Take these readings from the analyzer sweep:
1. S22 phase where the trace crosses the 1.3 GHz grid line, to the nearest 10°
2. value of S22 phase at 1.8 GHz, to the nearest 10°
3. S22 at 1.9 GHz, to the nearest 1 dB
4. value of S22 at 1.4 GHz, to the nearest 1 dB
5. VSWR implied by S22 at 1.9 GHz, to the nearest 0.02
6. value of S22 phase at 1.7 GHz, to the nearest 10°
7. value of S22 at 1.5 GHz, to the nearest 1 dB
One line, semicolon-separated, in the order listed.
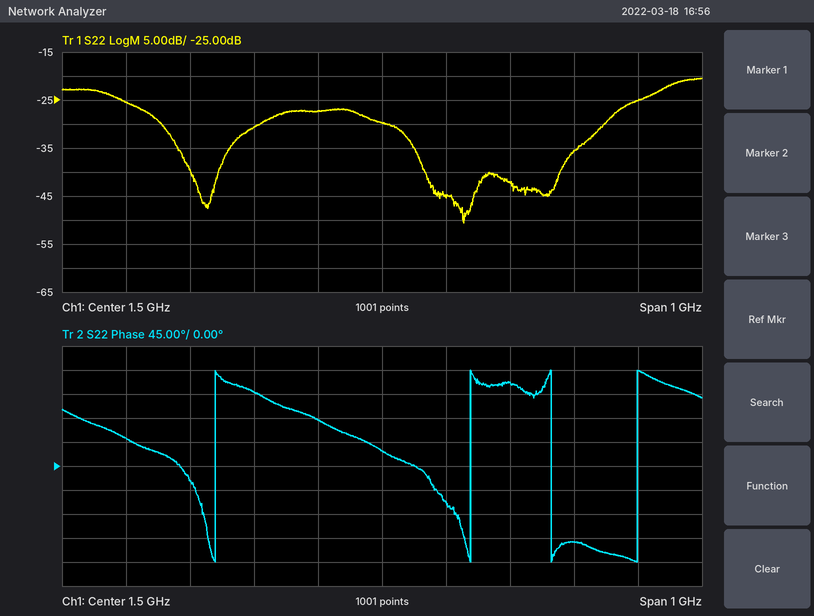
140°; -140°; -25 dB; -27 dB; 1.12; 160°; -30 dB
